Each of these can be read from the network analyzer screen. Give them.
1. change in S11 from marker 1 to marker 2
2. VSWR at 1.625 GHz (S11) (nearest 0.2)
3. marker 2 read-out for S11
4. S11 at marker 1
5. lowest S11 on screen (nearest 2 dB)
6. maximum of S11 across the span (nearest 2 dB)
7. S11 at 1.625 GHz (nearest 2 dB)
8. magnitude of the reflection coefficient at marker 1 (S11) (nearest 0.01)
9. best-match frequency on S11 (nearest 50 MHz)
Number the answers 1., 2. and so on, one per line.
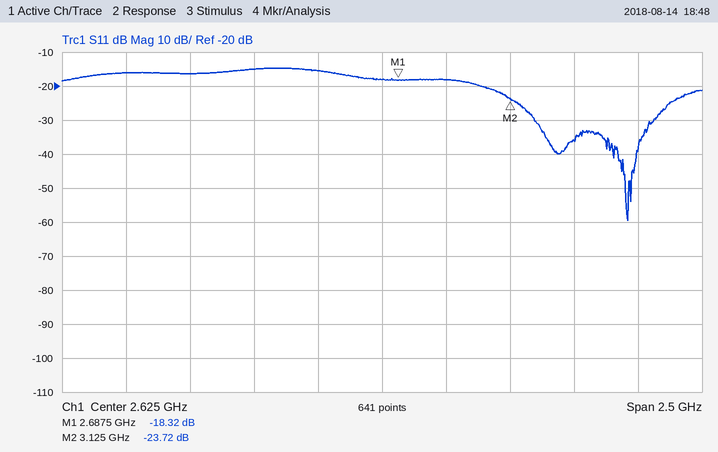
1. -5.40 dB
2. 1.4
3. -23.72 dB
4. -18.32 dB
5. -60 dB
6. -14 dB
7. -16 dB
8. 0.12
9. 3.60 GHz
